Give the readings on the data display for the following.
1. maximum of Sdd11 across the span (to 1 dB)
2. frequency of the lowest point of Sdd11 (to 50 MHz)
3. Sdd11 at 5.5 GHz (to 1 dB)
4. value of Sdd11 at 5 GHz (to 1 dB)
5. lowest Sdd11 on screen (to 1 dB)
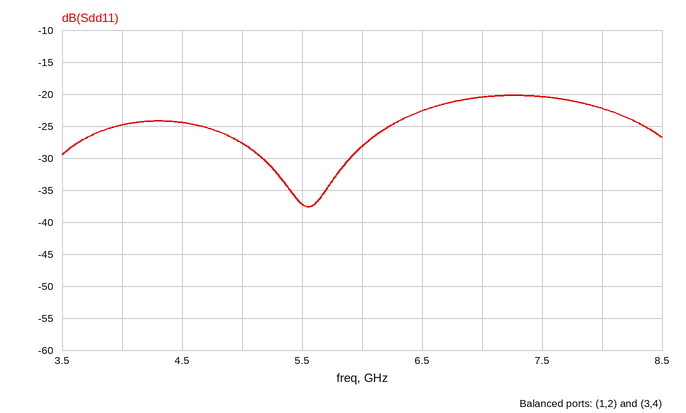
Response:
-20 dB
5.55 GHz
-37 dB
-28 dB
-38 dB
